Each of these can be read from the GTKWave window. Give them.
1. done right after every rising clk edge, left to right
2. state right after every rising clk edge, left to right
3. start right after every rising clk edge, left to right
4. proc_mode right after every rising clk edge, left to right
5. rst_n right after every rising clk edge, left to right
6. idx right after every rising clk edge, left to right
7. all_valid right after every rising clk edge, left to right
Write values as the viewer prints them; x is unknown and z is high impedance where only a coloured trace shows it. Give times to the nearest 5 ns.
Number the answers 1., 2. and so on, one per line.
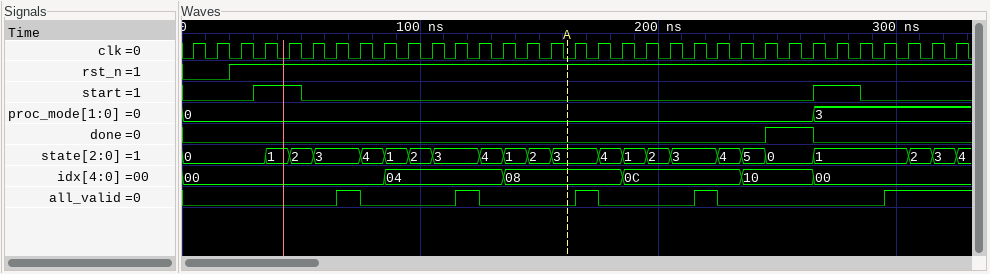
1. 0 0 0 0 0 0 0 0 0 0 0 0 0 0 0 0 0 0 0 0 0 0 0 0 1 1 0 0 0 0 0 0 0
2. 0, 0, 0, 1, 2, 3, 3, 4, 1, 2, 3, 3, 4, 1, 2, 3, 3, 4, 1, 2, 3, 3, 4, 5, 0, 0, 1, 1, 1, 1, 2, 3, 4
3. 0 0 0 1 1 0 0 0 0 0 0 0 0 0 0 0 0 0 0 0 0 0 0 0 0 0 1 1 0 0 0 0 0
4. 0, 0, 0, 0, 0, 0, 0, 0, 0, 0, 0, 0, 0, 0, 0, 0, 0, 0, 0, 0, 0, 0, 0, 0, 0, 0, 3, 3, 3, 3, 3, 3, 3
5. 0 0 1 1 1 1 1 1 1 1 1 1 1 1 1 1 1 1 1 1 1 1 1 1 1 1 1 1 1 1 1 1 1
6. 00, 00, 00, 00, 00, 00, 00, 00, 04, 04, 04, 04, 04, 08, 08, 08, 08, 08, 0C, 0C, 0C, 0C, 0C, 10, 10, 10, 00, 00, 00, 00, 00, 00, 00
7. 0 0 0 0 0 0 1 0 0 0 0 1 0 0 0 0 1 0 0 0 0 1 0 0 0 0 0 0 0 1 1 1 1
